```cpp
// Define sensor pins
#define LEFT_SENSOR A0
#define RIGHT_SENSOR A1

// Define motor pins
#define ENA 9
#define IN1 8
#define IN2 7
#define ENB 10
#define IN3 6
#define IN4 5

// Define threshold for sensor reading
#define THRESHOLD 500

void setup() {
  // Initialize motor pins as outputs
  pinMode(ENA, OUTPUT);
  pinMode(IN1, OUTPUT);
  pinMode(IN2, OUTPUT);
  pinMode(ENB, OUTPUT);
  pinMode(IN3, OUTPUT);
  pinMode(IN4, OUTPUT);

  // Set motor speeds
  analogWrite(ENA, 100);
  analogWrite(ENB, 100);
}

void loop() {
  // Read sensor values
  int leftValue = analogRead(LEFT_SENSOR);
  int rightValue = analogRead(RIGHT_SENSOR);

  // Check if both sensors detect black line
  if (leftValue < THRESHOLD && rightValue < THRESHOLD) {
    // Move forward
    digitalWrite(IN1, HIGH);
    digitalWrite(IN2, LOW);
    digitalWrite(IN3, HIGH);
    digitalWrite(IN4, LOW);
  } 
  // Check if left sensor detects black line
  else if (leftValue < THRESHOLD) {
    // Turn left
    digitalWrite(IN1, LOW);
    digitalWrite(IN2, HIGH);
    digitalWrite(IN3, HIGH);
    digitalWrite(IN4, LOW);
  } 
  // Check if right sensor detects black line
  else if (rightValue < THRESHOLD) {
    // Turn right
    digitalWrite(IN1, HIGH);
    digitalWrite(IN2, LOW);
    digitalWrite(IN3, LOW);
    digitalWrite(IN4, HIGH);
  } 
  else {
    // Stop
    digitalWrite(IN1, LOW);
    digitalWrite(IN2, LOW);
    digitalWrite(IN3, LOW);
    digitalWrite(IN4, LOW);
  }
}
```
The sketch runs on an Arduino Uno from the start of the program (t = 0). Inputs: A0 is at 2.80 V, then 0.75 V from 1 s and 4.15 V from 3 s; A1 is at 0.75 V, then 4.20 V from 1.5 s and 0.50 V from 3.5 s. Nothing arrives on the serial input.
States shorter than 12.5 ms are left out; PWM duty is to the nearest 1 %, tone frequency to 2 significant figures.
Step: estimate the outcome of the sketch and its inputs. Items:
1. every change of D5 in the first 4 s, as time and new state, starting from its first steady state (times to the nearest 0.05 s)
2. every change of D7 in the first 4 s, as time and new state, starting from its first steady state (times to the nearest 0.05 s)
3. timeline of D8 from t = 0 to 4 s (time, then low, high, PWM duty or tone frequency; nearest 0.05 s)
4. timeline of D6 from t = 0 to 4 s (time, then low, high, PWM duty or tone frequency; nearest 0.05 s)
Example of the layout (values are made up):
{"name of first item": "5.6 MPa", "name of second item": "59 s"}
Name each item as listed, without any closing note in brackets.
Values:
{"every change of D5 in the first 4 s, as time and new state, starting from its first steady state": "0 s high; 1 s low; 3.5 s high", "every change of D7 in the first 4 s, as time and new state, starting from its first steady state": "0 s low; 1.5 s high; 3 s low", "timeline of D8 from t = 0 to 4 s": "0 s high; 1.5 s low; 3.5 s high", "timeline of D6 from t = 0 to 4 s": "0 s low; 1 s high; 3 s low"}
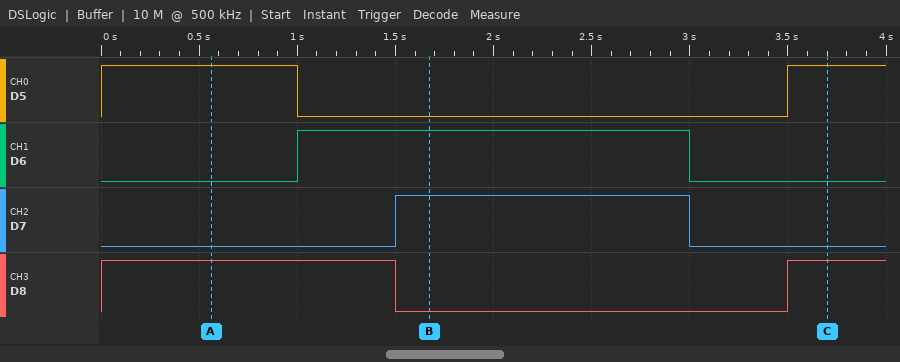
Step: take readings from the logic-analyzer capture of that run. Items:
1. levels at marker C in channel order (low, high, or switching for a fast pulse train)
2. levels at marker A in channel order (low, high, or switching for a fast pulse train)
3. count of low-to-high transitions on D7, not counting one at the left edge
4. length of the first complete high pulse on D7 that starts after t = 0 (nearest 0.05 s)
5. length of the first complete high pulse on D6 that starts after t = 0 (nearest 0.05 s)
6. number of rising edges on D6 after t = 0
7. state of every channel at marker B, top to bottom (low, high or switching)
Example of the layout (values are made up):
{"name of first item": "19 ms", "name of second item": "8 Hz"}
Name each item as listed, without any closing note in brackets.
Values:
{"levels at marker C in channel order": "D5 high, D6 low, D7 low, D8 high", "levels at marker A in channel order": "D5 high, D6 low, D7 low, D8 high", "count of low-to-high transitions on D7, not counting one at the left edge": "1", "length of the first complete high pulse on D7 that starts after t = 0": "1.50 s", "length of the first complete high pulse on D6 that starts after t = 0": "2.00 s", "number of rising edges on D6 after t = 0": "1", "state of every channel at marker B, top to bottom": "D5 low, D6 high, D7 high, D8 low"}
